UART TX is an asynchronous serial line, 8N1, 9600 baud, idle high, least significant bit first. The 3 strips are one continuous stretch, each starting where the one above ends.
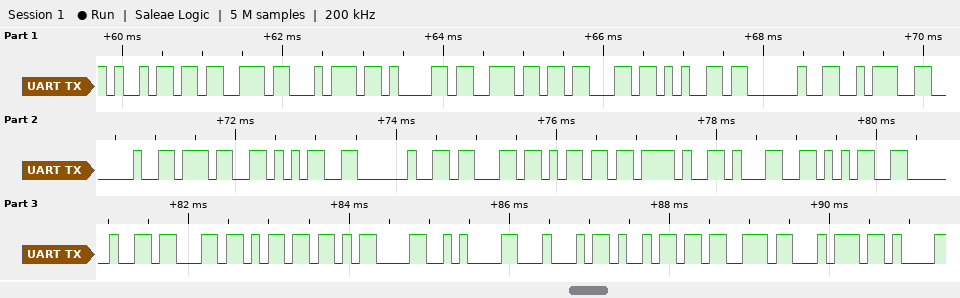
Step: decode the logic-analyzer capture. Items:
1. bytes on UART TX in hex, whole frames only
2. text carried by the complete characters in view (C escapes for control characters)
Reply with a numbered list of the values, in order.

1. 0x69 0x73 0x74 0x61 0x6E 0x63 0x65 0x20 0x3A 0x20 0x37 0x35 0x20 0x63 0x6D 0x2F 0x31 0x35 0x20 0x63 0x6D 0x0D 0x0A 0x44 0x69 0x73 0x74
2. "istance : 75 cm/15 cm\r\nDist"
